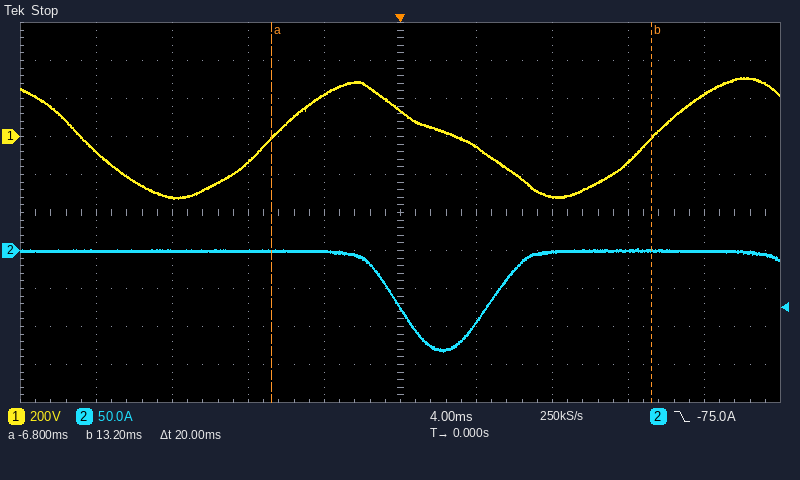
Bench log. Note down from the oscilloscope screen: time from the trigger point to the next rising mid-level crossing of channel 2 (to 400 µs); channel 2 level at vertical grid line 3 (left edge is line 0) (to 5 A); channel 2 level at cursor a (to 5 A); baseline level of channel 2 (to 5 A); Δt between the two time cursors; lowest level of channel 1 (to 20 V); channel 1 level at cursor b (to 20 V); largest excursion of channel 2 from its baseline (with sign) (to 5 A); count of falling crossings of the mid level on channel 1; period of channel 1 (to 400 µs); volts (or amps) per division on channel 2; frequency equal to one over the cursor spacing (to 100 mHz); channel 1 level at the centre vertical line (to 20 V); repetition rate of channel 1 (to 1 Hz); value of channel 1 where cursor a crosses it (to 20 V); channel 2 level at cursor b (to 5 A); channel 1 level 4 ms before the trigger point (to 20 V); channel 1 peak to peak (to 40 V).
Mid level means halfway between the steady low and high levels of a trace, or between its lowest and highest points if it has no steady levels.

4.8 ms
0 A
0 A
0 A
20 ms
-320 V
0 V
-130 A
2
20.0 ms
50 A
50.0 Hz
140 V
50 Hz
0 V
0 A
220 V
640 V
